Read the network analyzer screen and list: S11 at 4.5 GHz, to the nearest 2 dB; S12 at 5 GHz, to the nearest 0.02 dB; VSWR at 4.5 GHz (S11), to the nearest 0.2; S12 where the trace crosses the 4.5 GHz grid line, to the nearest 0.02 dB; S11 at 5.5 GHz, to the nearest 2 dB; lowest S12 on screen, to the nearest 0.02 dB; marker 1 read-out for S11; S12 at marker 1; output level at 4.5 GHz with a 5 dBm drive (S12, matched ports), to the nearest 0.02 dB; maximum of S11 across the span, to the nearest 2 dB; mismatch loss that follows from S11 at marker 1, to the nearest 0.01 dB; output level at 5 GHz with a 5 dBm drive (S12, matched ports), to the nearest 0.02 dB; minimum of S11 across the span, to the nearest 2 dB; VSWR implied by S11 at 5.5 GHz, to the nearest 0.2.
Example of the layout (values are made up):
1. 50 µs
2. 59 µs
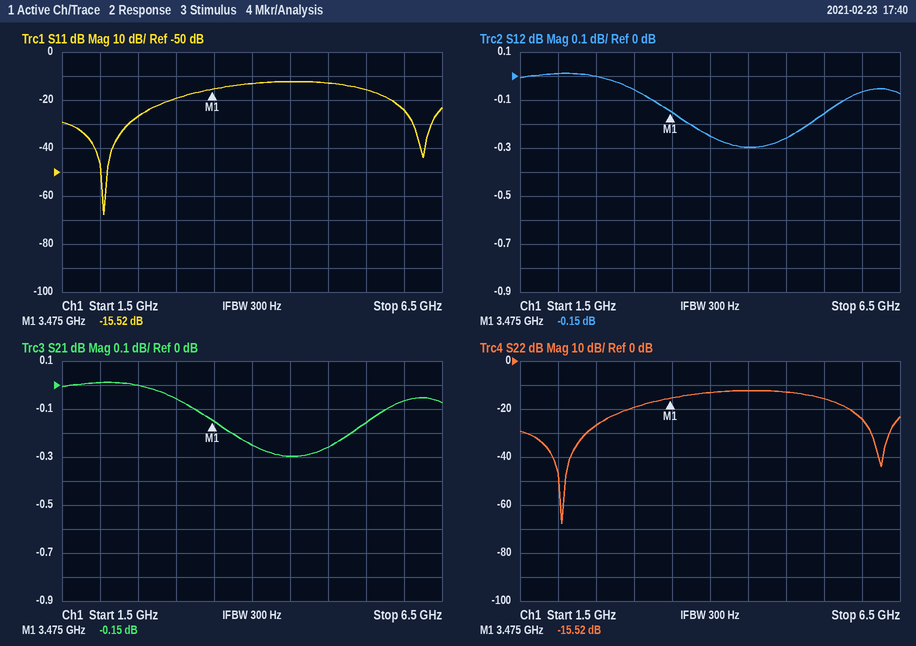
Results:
1. -12 dB
2. -0.26 dB
3. 1.6
4. -0.30 dB
5. -16 dB
6. -0.30 dB
7. -15.52 dB
8. -0.15 dB
9. 4.70 dBm
10. -12 dB
11. 0.12 dB
12. 4.74 dBm
13. -68 dB
14. 1.4
